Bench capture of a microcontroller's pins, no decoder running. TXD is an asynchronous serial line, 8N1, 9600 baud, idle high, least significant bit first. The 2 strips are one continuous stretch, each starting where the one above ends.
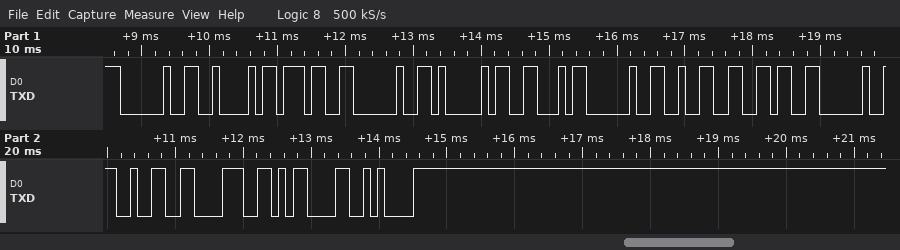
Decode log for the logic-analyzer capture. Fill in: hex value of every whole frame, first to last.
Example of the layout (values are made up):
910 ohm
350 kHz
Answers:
0x20 0x42 0x37 0x20 0x41 0x46 0x20 0x32 0x36 0x20 0x32 0x38 0x0D 0x0A
